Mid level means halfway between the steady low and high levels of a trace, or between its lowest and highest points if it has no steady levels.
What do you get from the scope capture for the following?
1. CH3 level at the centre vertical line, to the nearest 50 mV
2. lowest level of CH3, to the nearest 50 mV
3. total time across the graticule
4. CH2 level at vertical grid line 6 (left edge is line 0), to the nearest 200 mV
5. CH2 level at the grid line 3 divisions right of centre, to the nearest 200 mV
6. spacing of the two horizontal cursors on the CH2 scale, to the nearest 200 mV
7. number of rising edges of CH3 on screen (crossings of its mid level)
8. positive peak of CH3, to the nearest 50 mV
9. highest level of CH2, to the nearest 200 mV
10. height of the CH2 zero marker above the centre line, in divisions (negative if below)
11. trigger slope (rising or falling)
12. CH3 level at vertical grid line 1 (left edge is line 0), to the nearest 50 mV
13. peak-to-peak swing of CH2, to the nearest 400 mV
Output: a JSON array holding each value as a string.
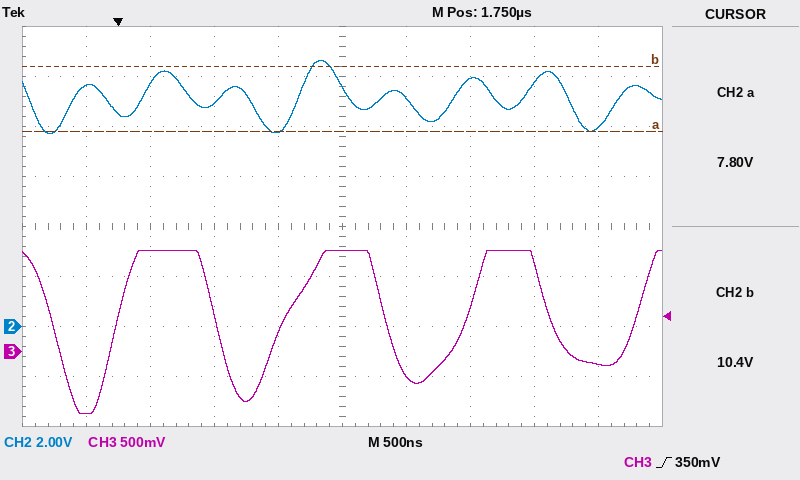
["1.00 V", "-600 mV", "5 µs", "9.2 V", "9.8 V", "2.6 V", "4", "1.00 V", "10.6 V", "-2.0 div", "rising", "-600 mV", "2.8 V"]
